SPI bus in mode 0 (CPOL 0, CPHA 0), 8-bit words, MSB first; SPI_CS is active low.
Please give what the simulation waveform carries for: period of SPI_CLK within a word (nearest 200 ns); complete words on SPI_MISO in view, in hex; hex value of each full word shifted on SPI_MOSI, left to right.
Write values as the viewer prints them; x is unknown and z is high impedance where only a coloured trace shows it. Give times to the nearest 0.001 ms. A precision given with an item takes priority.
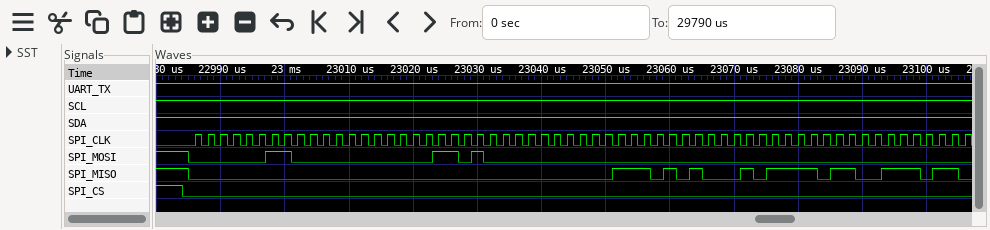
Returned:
2000 ns
00, 00, 00, 00, 75, 17, B3
03, 00, 1A, 00, 00, 00, 00
